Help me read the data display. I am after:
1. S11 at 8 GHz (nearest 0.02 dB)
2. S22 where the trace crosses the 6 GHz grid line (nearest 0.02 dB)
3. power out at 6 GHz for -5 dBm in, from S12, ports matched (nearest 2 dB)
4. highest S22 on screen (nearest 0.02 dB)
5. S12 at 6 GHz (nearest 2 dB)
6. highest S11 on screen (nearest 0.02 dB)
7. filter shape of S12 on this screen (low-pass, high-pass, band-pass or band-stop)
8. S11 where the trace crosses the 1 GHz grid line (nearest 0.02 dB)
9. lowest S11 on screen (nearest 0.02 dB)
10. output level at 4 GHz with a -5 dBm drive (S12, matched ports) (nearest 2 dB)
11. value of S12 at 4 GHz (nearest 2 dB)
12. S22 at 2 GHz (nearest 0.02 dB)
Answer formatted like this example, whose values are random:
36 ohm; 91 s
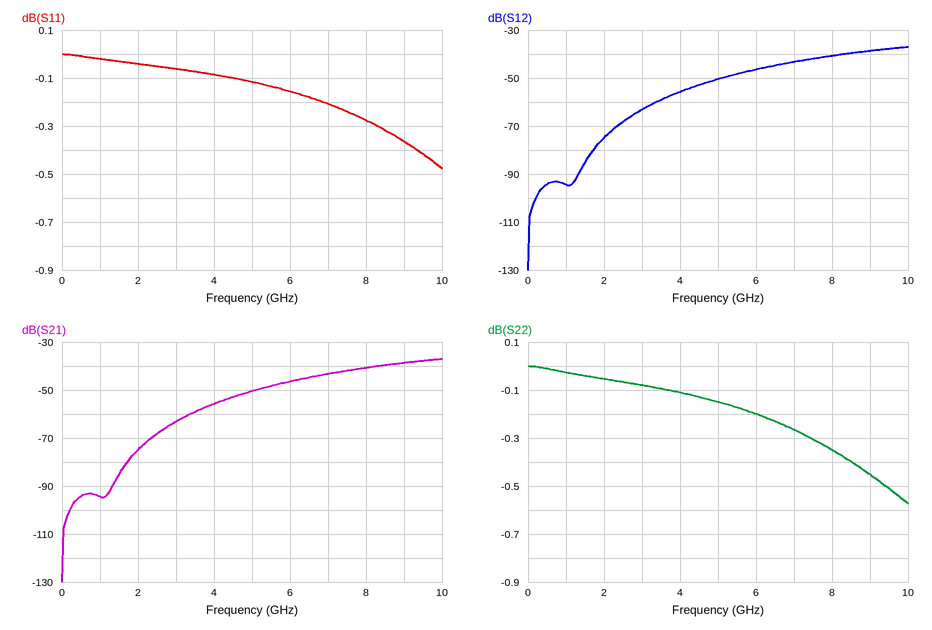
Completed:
-0.28 dB; -0.20 dB; -52 dBm; 0.00 dB; -46 dB; 0.00 dB; high-pass; -0.02 dB; -0.48 dB; -60 dBm; -56 dB; -0.06 dB
